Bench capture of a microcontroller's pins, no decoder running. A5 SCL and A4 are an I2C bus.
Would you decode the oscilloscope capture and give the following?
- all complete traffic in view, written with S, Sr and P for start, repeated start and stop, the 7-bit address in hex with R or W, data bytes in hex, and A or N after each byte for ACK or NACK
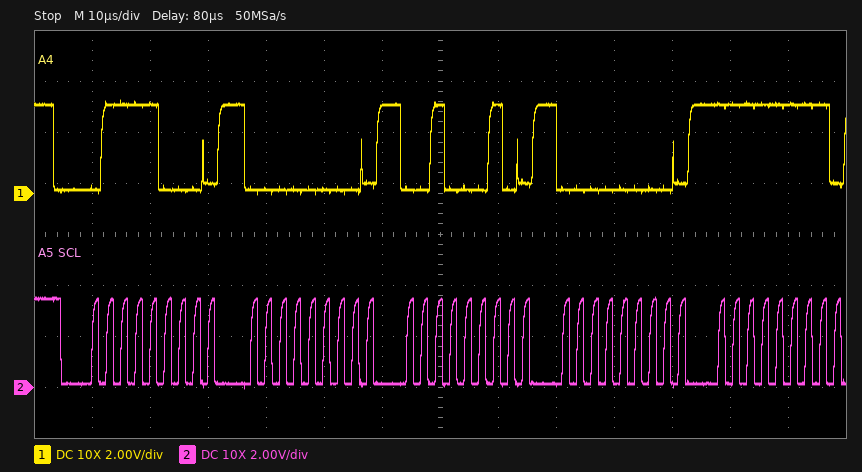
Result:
S 3CW A 00 A 22 A 00 A FF A
